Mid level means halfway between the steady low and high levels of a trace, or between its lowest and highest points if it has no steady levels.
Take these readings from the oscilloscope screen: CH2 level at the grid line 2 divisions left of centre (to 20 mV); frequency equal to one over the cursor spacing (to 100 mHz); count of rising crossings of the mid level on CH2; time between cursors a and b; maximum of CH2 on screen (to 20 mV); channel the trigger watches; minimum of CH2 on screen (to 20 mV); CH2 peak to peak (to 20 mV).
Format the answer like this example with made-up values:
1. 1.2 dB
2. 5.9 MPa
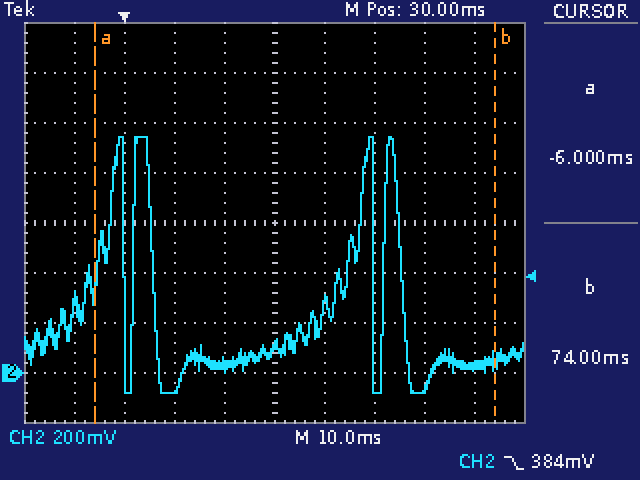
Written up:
1. -60 mV
2. 12.5 Hz
3. 4
4. 80 ms
5. 940 mV
6. CH2
7. -80 mV
8. 1.02 V
